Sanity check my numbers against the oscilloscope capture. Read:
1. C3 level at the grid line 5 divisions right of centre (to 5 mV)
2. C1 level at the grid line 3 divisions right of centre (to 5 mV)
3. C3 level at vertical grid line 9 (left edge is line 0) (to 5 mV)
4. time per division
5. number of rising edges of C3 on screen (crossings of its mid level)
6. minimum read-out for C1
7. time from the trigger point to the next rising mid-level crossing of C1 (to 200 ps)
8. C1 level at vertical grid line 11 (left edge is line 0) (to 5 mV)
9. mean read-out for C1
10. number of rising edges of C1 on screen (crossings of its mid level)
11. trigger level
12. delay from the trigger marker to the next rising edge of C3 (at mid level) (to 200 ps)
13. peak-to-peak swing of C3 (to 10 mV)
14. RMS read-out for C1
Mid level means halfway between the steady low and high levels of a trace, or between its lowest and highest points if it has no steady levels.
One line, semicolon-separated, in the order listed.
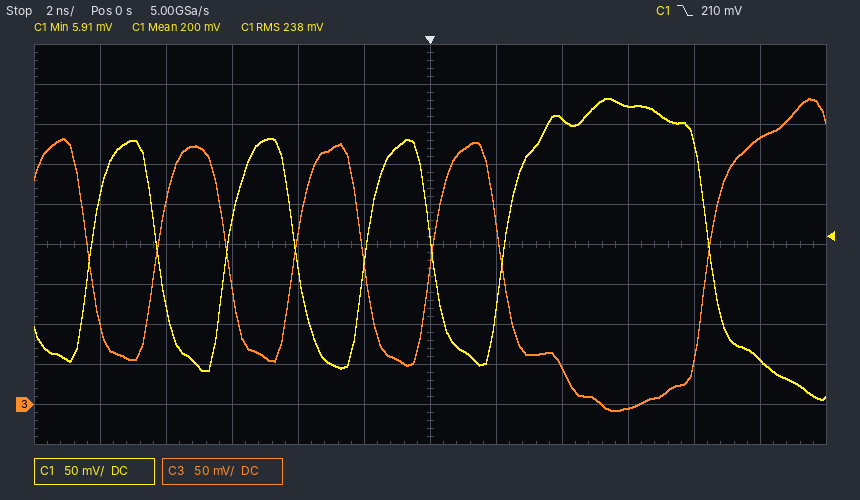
335 mV; 375 mV; -5 mV; 2 ns; 4; 5.91 mV; 2.2 ns; 55 mV; 200 mV; 4; 210 mV; 8.4 ns; 390 mV; 238 mV
